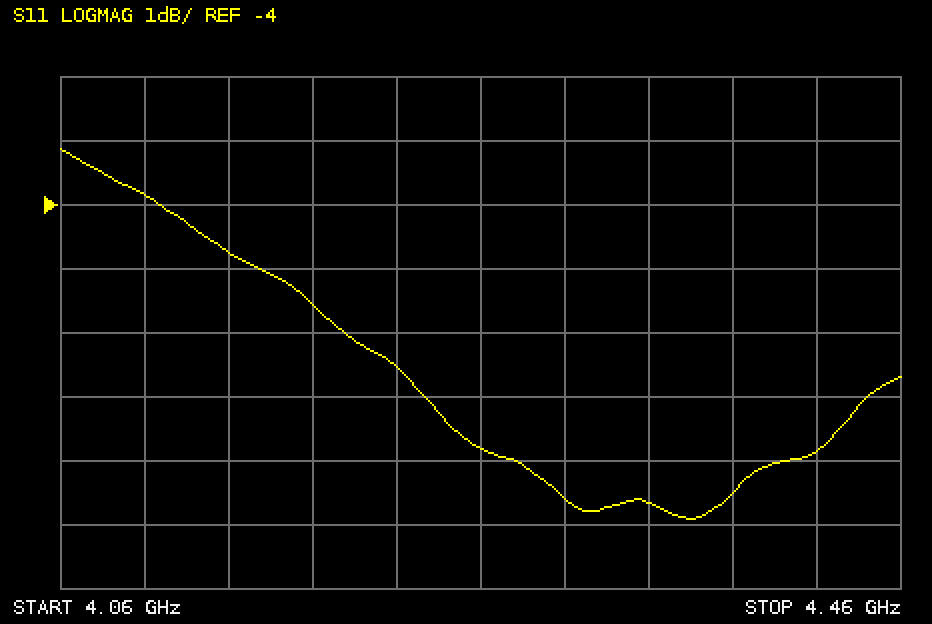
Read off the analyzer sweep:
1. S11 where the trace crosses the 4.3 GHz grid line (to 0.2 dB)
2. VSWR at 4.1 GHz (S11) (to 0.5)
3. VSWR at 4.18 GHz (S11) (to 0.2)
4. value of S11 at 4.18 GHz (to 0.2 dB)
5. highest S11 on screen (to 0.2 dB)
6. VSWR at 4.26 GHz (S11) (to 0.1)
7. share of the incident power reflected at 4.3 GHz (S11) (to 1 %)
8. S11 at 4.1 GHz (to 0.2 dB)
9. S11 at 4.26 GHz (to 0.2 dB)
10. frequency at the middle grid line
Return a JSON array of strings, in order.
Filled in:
["-8.6 dB", "4.5", "3.2", "-5.6 dB", "-3.2 dB", "2.4", "14 %", "-3.8 dB", "-7.8 dB", "4.26 GHz"]
